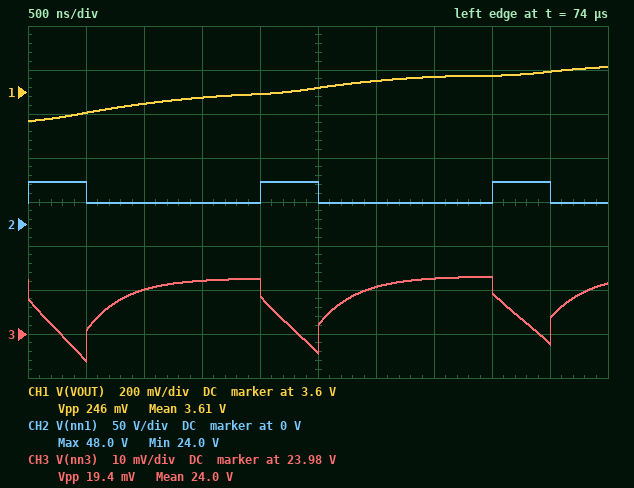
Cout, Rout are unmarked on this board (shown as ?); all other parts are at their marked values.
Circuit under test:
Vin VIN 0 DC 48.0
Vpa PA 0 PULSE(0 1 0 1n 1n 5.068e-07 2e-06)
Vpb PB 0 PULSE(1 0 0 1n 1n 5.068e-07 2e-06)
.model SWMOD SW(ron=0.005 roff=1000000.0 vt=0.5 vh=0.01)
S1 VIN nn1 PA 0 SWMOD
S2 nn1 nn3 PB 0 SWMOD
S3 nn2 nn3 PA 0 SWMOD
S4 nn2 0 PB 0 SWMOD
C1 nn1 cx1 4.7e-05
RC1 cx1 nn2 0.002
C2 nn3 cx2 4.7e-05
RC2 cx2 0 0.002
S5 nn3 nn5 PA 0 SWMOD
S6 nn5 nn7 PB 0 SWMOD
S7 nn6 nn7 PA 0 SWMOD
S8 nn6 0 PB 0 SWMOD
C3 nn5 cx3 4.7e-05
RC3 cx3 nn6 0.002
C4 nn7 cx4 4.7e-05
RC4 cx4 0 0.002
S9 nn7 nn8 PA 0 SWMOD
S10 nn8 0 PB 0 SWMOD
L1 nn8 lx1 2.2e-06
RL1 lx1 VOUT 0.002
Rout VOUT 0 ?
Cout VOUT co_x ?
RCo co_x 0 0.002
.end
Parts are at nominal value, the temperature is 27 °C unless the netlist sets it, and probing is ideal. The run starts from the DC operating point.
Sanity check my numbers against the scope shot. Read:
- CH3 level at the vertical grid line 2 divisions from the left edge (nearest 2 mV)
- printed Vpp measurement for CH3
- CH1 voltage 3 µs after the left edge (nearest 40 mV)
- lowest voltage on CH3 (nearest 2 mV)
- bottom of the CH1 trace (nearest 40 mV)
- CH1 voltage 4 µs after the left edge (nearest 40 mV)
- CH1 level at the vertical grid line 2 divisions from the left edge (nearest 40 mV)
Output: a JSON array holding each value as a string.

["23.990 V", "19.4 mV", "3.64 V", "23.974 V", "3.48 V", "3.68 V", "3.56 V"]
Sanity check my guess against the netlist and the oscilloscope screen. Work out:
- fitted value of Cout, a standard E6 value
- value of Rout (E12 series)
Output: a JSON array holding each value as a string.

["33 µF", "1 Ω"]
